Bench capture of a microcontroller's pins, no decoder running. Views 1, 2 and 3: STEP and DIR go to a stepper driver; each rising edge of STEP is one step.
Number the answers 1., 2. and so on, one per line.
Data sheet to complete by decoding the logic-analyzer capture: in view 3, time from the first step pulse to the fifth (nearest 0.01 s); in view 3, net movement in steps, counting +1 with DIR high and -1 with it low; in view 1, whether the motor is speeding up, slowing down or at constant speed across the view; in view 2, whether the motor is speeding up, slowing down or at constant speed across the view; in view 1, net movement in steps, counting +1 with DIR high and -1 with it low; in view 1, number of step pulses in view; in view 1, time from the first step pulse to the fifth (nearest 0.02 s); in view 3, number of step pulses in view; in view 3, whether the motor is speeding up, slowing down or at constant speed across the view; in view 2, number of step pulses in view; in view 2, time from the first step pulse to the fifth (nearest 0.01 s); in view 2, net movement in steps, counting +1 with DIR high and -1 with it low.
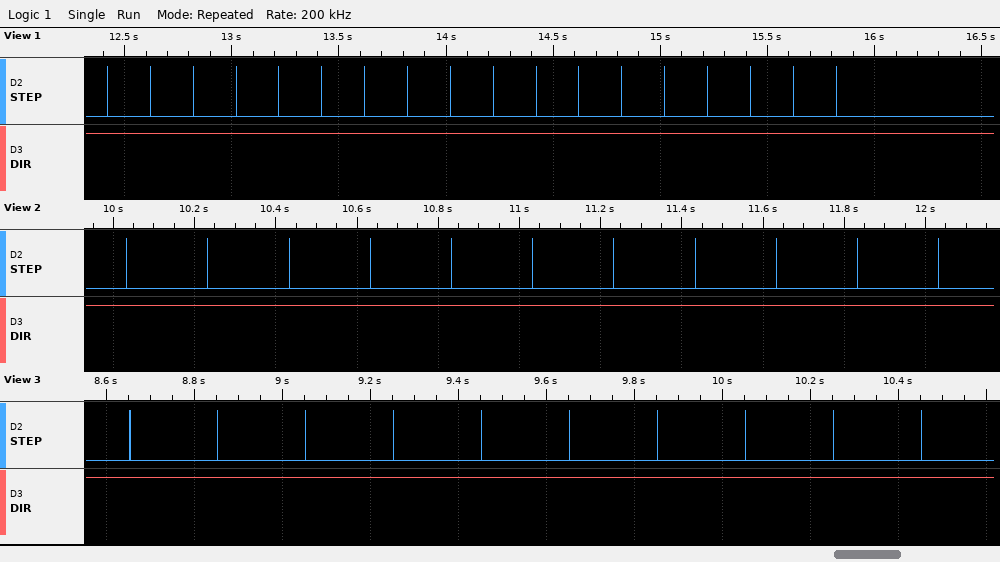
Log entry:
1. 0.80 s
2. +10
3. constant speed
4. constant speed
5. +18
6. 18
7. 0.80 s
8. 10
9. constant speed
10. 11
11. 0.80 s
12. +11
